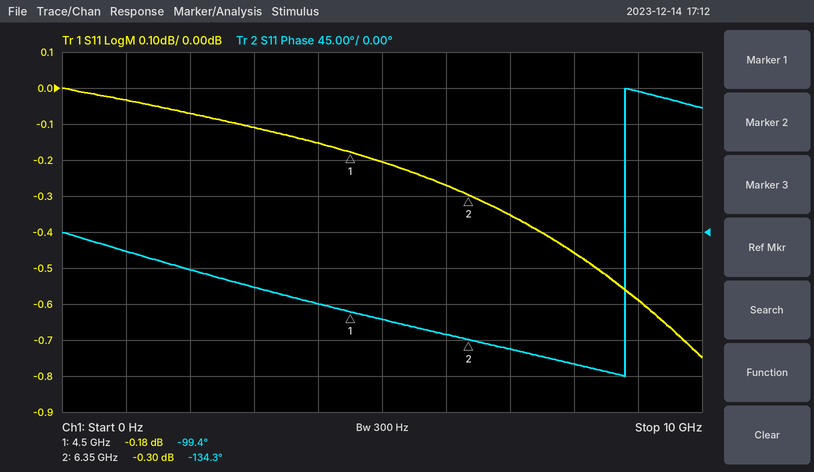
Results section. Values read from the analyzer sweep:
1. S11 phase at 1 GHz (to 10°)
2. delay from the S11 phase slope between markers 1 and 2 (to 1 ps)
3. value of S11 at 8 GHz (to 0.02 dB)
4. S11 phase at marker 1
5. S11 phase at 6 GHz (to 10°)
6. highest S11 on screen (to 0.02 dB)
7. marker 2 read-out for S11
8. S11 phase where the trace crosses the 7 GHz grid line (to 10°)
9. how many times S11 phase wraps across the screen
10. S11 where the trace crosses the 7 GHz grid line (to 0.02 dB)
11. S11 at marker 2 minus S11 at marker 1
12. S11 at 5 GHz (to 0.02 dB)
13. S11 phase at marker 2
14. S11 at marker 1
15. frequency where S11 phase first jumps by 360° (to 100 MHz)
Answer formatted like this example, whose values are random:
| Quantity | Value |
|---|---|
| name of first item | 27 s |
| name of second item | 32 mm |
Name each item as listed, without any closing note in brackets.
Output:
| Quantity | Value |
|---|---|
| S11 phase at 1 GHz | -20° |
| delay from the S11 phase slope between markers 1 and 2 | 52 ps |
| value of S11 at 8 GHz | -0.46 dB |
| S11 phase at marker 1 | -99.4° |
| S11 phase at 6 GHz | -130° |
| highest S11 on screen | 0.00 dB |
| marker 2 read-out for S11 | -0.30 dB |
| S11 phase where the trace crosses the 7 GHz grid line | -150° |
| how many times S11 phase wraps across the screen | 1 |
| S11 where the trace crosses the 7 GHz grid line | -0.36 dB |
| S11 at marker 2 minus S11 at marker 1 | -0.12 dB |
| S11 at 5 GHz | -0.20 dB |
| S11 phase at marker 2 | -134.3° |
| S11 at marker 1 | -0.18 dB |
| frequency where S11 phase first jumps by 360° | 8.8 GHz |
